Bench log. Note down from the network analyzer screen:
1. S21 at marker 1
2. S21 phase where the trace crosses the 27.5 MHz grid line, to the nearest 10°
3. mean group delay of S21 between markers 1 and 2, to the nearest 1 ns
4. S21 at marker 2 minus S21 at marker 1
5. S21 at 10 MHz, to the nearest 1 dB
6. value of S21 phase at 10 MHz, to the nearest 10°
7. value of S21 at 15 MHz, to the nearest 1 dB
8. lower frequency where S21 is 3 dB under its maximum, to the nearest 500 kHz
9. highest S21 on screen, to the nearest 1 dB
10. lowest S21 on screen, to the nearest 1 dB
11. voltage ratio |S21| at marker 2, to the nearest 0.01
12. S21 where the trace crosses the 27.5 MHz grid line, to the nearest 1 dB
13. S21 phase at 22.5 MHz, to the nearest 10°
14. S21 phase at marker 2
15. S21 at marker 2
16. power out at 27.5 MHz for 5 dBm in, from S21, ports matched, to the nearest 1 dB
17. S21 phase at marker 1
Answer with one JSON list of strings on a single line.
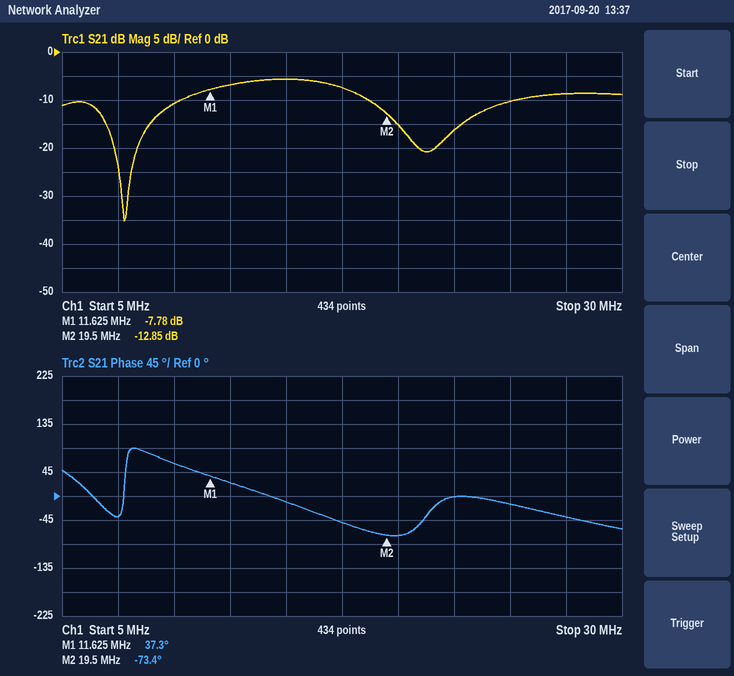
["-7.78 dB", "-40°", "39 ns", "-5.07 dB", "-11 dB", "60°", "-6 dB", "11.0 MHz", "-6 dB", "-35 dB", "0.23", "-9 dB", "0°", "-73.4°", "-12.85 dB", "-4 dBm", "37.3°"]
